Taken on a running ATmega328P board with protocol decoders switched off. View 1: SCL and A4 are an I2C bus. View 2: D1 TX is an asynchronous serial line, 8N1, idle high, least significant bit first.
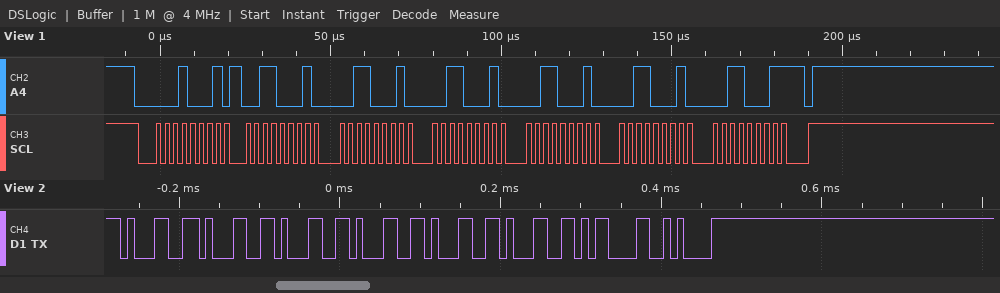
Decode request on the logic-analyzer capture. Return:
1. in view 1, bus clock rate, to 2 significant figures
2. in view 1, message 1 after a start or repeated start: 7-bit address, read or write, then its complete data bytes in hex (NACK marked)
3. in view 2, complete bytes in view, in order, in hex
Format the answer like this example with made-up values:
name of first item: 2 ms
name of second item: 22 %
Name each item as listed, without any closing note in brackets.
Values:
in view 1, bus clock rate, to 2 significant figures: 400 kHz
in view 1, message 1 after a start or repeated start: 7-bit address, read or write, then its complete data bytes in hex: 0x08 read: 31 31 31 31 31 31 NACK
in view 2, complete bytes in view, in order, in hex: 31 31 31 31 31 31 0D 0A
